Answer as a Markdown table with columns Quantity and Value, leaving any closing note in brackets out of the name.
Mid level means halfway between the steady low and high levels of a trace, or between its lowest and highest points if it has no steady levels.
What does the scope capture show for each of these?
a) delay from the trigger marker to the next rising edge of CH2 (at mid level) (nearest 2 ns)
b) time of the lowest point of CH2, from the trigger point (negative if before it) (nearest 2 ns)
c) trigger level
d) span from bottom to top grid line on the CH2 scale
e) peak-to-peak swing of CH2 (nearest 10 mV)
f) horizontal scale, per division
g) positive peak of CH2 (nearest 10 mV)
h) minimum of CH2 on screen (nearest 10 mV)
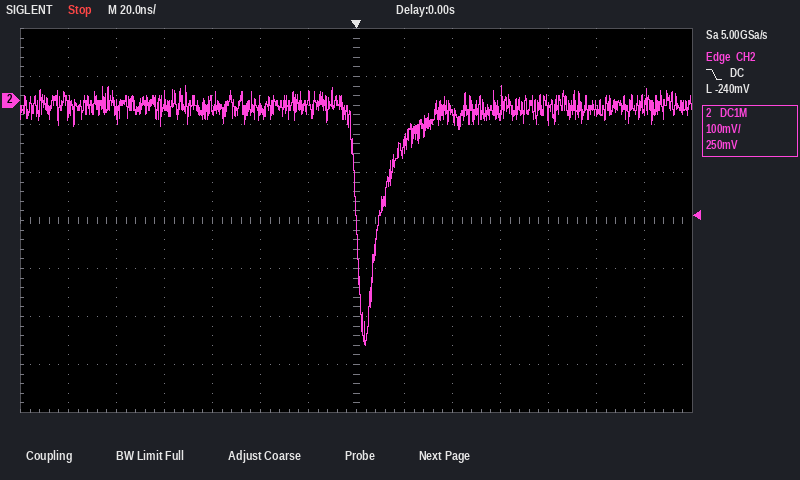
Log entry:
| Quantity | Value |
|---|---|
| delay from the trigger marker to the next rising edge of CH2 (at mid level) | 10 ns |
| time of the lowest point of CH2, from the trigger point (negative if before it) | +4 ns |
| trigger level | -240 mV |
| span from bottom to top grid line on the CH2 scale | 800 mV |
| peak-to-peak swing of CH2 | 540 mV |
| horizontal scale, per division | 20 ns |
| positive peak of CH2 | 30 mV |
| minimum of CH2 on screen | -510 mV |
